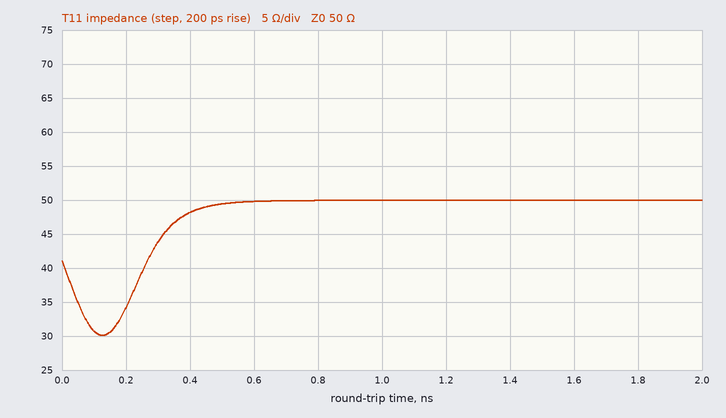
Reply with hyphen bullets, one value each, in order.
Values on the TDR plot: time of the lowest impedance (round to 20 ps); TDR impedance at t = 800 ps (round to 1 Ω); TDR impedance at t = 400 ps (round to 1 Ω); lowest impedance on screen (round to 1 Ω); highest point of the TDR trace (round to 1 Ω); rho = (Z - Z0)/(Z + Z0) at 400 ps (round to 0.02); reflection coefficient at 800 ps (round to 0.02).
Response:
- 120 ps
- 50 Ω
- 48 Ω
- 30 Ω
- 50 Ω
- -0.02
- 0.00
